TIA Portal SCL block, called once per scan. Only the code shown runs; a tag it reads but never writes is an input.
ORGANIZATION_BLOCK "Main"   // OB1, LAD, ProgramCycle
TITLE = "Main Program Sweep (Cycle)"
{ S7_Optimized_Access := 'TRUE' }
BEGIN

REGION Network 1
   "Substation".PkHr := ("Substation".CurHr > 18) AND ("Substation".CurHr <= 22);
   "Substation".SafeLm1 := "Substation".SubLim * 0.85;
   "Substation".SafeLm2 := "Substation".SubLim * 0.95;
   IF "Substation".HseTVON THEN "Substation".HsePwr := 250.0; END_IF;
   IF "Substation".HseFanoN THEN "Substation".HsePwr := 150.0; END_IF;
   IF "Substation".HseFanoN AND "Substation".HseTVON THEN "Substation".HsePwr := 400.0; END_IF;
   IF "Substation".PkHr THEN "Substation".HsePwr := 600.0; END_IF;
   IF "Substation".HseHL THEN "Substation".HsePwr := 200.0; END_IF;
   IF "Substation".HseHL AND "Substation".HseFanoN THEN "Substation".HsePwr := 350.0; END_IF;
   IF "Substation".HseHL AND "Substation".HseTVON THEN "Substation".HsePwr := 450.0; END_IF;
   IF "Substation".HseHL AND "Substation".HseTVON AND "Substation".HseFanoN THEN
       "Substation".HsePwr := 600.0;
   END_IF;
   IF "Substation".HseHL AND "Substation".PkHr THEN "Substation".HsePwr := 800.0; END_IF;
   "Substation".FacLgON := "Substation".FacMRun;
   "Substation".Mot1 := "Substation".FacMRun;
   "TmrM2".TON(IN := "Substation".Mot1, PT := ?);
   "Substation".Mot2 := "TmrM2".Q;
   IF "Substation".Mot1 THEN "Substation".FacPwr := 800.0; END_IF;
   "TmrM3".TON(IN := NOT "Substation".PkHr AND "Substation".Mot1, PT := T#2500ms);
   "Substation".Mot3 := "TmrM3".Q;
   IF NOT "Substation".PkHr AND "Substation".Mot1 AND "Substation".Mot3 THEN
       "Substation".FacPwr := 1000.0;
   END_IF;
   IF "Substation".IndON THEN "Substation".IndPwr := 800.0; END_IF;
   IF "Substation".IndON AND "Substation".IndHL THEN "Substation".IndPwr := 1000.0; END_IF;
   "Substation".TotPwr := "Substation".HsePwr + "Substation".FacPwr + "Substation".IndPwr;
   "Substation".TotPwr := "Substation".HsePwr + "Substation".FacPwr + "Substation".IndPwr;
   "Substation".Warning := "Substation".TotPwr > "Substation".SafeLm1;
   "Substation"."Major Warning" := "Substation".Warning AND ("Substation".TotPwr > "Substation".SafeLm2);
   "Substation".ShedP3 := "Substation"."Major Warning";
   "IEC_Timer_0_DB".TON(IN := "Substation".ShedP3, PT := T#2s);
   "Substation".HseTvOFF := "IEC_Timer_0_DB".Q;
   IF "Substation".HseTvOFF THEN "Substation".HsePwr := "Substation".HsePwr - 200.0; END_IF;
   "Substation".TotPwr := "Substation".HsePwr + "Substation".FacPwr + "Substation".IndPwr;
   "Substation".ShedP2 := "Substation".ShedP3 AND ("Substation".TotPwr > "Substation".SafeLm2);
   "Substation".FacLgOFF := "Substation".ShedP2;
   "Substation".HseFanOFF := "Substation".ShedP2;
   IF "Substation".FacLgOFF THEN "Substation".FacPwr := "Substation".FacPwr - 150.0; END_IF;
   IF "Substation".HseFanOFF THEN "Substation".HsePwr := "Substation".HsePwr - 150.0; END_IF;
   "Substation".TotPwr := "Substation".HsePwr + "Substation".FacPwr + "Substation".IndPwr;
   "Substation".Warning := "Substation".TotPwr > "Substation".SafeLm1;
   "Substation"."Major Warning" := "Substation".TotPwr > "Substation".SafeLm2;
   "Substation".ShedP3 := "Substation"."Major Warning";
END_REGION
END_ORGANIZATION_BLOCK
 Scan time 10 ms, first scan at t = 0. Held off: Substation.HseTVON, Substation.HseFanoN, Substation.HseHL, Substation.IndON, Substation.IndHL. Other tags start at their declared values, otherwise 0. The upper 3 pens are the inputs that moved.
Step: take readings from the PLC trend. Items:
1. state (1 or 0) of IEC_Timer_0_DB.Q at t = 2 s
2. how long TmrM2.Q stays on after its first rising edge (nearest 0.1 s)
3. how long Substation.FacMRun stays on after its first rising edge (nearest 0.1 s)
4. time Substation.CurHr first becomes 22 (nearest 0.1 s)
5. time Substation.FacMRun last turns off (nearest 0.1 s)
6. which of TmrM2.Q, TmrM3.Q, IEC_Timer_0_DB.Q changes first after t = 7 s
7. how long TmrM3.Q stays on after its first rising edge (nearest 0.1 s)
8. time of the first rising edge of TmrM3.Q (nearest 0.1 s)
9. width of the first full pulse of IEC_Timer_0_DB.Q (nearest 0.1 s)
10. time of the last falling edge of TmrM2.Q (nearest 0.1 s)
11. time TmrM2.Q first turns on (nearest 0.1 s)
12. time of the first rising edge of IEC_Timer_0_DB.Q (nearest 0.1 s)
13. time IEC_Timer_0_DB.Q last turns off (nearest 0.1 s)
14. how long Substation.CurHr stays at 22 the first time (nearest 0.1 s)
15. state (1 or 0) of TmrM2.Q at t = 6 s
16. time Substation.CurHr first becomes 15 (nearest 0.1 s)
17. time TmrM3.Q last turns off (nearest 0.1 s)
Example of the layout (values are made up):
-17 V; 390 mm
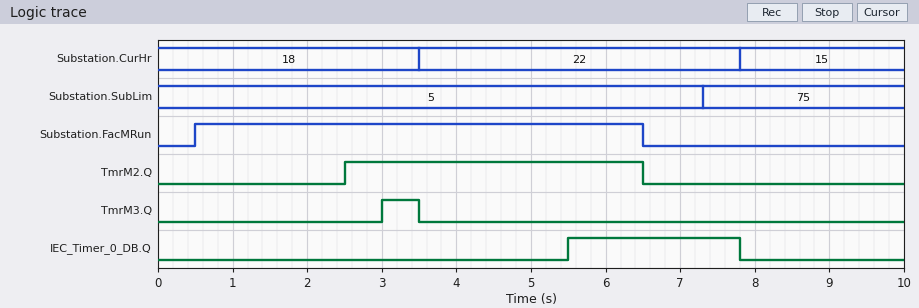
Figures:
0; 4.0 s; 6.0 s; 3.5 s; 6.5 s; IEC_Timer_0_DB.Q; 0.5 s; 3.0 s; 2.3 s; 6.5 s; 2.5 s; 5.5 s; 7.8 s; 4.3 s; 1; 7.8 s; 3.5 s
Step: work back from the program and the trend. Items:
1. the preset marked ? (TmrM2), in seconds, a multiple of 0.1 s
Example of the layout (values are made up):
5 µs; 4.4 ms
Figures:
2.0 s
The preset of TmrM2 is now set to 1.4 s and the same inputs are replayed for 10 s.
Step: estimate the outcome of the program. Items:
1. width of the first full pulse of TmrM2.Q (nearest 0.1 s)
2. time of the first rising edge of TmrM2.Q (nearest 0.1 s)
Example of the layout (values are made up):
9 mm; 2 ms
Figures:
4.6 s; 1.9 s
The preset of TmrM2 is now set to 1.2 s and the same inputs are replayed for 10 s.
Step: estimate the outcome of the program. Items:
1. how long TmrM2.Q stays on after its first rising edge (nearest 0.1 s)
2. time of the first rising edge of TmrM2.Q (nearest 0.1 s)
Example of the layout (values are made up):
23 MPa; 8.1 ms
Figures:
4.8 s; 1.7 s
